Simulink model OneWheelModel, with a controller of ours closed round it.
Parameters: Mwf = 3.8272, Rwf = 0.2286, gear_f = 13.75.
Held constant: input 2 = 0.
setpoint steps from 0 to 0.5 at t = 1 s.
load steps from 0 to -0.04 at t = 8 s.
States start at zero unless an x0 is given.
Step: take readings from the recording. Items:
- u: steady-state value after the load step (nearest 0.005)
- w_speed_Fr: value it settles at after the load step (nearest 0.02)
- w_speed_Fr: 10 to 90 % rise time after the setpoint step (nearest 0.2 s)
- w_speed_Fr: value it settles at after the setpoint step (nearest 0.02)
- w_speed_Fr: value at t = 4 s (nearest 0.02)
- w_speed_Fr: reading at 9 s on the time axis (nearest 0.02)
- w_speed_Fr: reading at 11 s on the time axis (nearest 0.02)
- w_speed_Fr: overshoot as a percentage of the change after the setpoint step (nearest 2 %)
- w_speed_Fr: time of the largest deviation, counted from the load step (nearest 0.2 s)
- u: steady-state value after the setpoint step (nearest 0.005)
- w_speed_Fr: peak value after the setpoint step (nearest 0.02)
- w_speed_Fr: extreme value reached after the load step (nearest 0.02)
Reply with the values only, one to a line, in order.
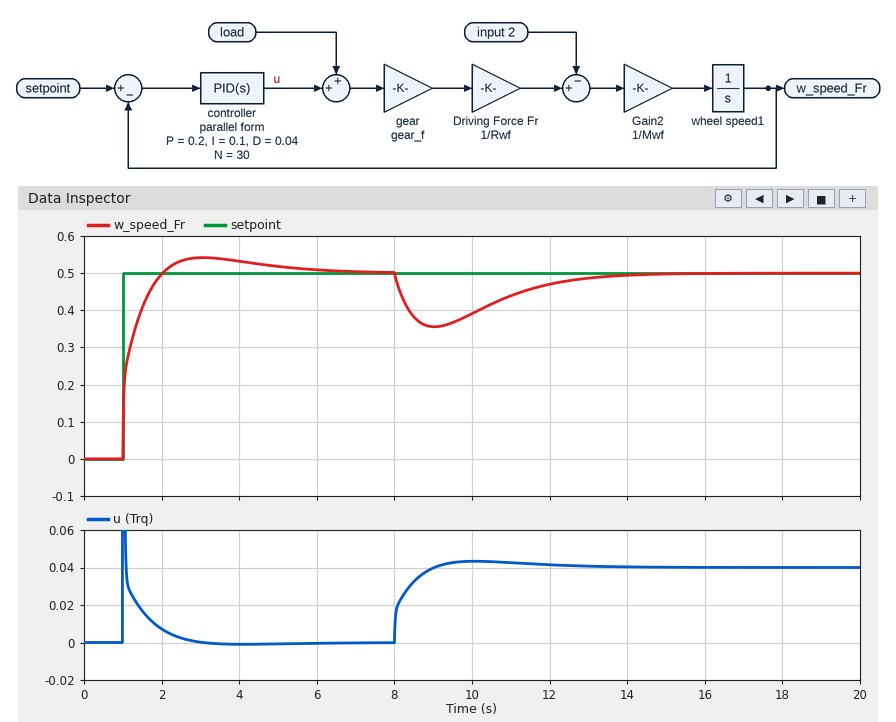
0.040
0.50
0.6 s
0.50
0.54
0.36
0.44
8 %
1.0 s
0.000
0.54
0.36
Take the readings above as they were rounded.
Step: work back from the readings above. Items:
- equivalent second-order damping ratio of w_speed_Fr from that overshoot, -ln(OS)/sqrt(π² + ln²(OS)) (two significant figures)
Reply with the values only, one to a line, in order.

0.63
